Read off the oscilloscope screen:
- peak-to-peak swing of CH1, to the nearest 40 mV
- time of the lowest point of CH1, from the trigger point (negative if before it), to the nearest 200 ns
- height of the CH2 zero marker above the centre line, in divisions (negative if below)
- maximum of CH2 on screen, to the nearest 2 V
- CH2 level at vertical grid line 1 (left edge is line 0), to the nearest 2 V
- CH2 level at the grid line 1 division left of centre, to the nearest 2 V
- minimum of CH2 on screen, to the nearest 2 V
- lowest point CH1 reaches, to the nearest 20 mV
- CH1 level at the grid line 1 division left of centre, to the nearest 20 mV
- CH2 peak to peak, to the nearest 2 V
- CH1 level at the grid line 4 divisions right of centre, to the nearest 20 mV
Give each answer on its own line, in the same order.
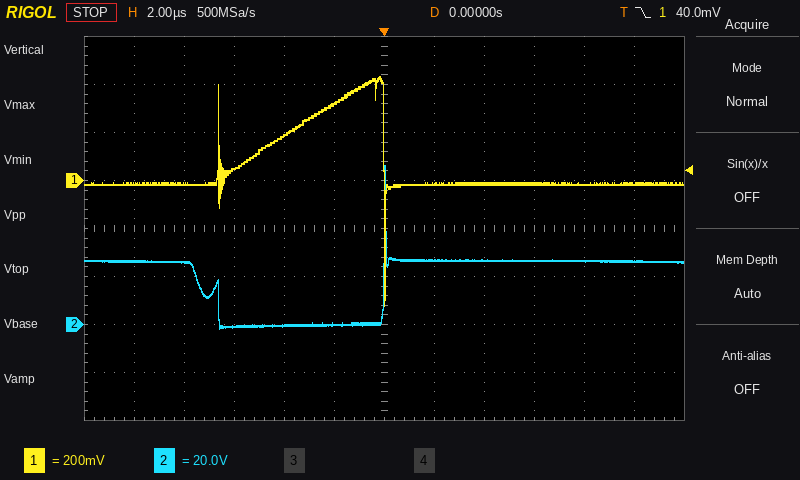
960 mV
0.0 µs
-2.0 div
66 V
26 V
0 V
-2 V
-520 mV
320 mV
68 V
-20 mV
